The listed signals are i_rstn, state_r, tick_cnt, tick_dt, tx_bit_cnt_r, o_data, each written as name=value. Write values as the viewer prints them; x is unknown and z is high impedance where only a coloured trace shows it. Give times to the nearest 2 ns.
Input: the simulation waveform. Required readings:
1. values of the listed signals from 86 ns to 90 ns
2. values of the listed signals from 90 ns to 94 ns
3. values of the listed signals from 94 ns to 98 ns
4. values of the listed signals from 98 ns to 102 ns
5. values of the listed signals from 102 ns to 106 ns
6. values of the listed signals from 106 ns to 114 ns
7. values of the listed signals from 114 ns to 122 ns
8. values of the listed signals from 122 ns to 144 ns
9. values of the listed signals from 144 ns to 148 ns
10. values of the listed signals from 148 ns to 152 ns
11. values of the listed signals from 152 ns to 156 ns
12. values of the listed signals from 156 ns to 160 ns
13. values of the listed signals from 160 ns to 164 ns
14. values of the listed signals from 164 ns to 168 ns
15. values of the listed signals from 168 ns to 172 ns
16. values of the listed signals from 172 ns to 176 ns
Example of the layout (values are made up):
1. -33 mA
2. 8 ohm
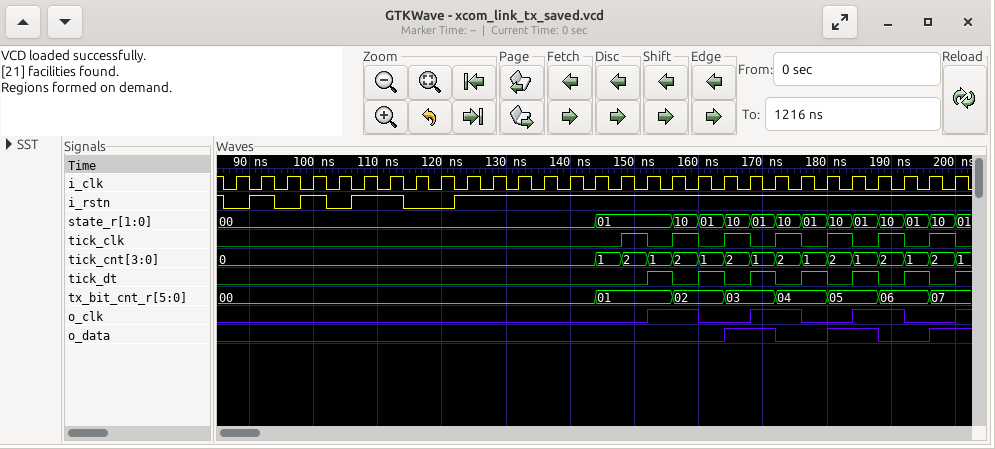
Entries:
1. i_rstn=0, state_r=00, tick_cnt=0, tick_dt=0, tx_bit_cnt_r=00, o_data=0
2. i_rstn=1, state_r=00, tick_cnt=0, tick_dt=0, tx_bit_cnt_r=00, o_data=0
3. i_rstn=0, state_r=00, tick_cnt=0, tick_dt=0, tx_bit_cnt_r=00, o_data=0
4. i_rstn=1, state_r=00, tick_cnt=0, tick_dt=0, tx_bit_cnt_r=00, o_data=0
5. i_rstn=0, state_r=00, tick_cnt=0, tick_dt=0, tx_bit_cnt_r=00, o_data=0
6. i_rstn=1, state_r=00, tick_cnt=0, tick_dt=0, tx_bit_cnt_r=00, o_data=0
7. i_rstn=0, state_r=00, tick_cnt=0, tick_dt=0, tx_bit_cnt_r=00, o_data=0
8. i_rstn=1, state_r=00, tick_cnt=0, tick_dt=0, tx_bit_cnt_r=00, o_data=0
9. i_rstn=1, state_r=01, tick_cnt=1, tick_dt=0, tx_bit_cnt_r=01, o_data=0
10. i_rstn=1, state_r=01, tick_cnt=2, tick_dt=0, tx_bit_cnt_r=01, o_data=0
11. i_rstn=1, state_r=01, tick_cnt=1, tick_dt=1, tx_bit_cnt_r=01, o_data=0
12. i_rstn=1, state_r=10, tick_cnt=2, tick_dt=0, tx_bit_cnt_r=02, o_data=0
13. i_rstn=1, state_r=01, tick_cnt=1, tick_dt=1, tx_bit_cnt_r=02, o_data=0
14. i_rstn=1, state_r=10, tick_cnt=2, tick_dt=0, tx_bit_cnt_r=03, o_data=1
15. i_rstn=1, state_r=01, tick_cnt=1, tick_dt=1, tx_bit_cnt_r=03, o_data=1
16. i_rstn=1, state_r=10, tick_cnt=2, tick_dt=0, tx_bit_cnt_r=04, o_data=0
